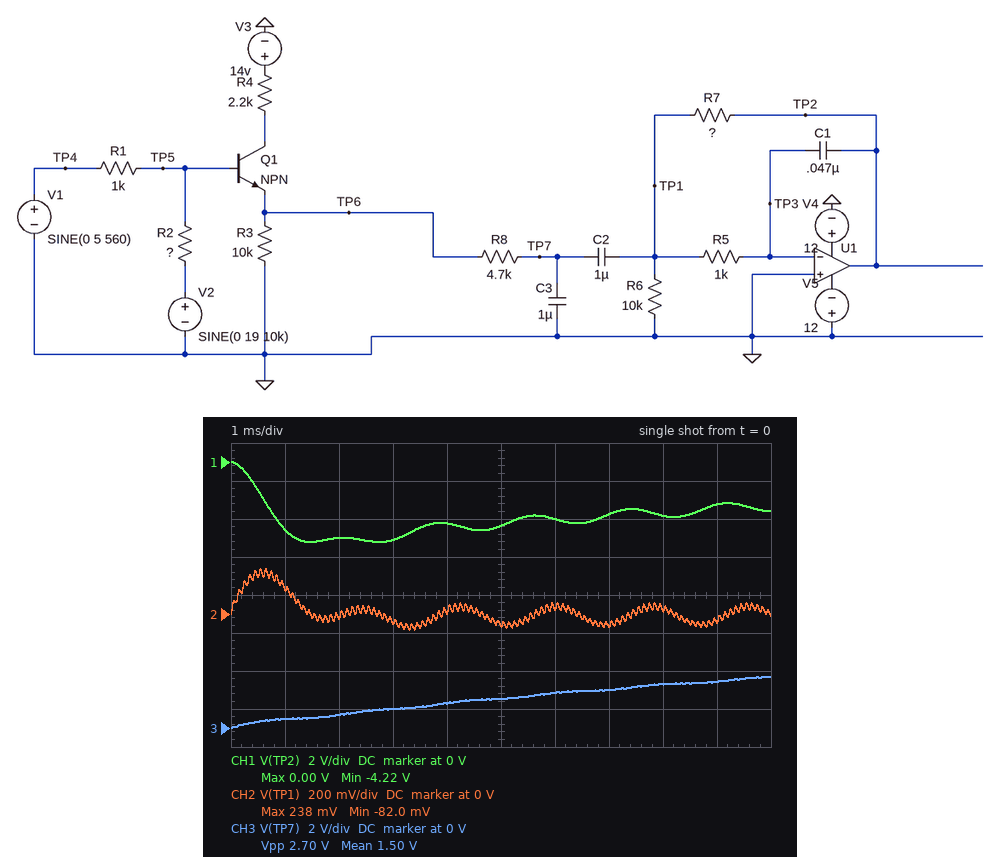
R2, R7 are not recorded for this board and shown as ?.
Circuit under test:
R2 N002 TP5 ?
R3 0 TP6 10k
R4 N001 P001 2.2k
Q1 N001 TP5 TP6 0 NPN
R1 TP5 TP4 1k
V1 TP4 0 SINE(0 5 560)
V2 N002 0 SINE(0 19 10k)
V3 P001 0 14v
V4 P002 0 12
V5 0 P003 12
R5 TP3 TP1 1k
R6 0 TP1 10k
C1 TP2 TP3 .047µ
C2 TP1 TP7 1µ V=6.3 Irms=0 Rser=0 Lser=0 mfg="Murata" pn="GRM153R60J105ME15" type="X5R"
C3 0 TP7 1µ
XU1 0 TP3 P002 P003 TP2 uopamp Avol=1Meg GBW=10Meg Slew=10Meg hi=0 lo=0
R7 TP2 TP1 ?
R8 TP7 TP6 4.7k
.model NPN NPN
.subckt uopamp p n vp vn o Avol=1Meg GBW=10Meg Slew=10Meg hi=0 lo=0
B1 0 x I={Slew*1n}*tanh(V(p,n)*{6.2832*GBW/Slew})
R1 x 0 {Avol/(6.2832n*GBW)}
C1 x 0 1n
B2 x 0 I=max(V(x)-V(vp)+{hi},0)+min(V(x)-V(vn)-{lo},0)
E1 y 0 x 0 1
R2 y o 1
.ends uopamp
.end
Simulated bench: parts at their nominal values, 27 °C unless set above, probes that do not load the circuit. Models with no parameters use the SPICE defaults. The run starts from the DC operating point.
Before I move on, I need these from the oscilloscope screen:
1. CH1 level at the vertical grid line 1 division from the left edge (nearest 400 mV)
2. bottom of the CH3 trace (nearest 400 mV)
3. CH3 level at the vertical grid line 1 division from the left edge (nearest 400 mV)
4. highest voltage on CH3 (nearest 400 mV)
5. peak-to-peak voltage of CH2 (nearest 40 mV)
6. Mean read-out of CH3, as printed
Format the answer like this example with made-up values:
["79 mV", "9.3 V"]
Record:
["-3.6 V", "0 V", "400 mV", "2.8 V", "320 mV", "1.50 V"]
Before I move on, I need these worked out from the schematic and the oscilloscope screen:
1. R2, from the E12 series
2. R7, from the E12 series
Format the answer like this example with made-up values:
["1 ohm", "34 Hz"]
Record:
["560 Ω", "12 kΩ"]
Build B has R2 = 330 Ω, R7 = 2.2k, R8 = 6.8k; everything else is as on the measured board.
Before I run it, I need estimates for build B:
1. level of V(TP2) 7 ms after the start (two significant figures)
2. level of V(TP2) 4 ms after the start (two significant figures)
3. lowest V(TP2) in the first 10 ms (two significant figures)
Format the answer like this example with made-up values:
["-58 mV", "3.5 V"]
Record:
["-340 mV", "-600 mV", "-930 mV"]
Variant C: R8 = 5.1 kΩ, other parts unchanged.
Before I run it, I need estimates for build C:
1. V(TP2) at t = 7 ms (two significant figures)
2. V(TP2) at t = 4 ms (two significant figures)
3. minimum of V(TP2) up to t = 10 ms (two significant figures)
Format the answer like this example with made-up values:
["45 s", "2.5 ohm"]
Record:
["-2.6 V", "-3.0 V", "-3.9 V"]
